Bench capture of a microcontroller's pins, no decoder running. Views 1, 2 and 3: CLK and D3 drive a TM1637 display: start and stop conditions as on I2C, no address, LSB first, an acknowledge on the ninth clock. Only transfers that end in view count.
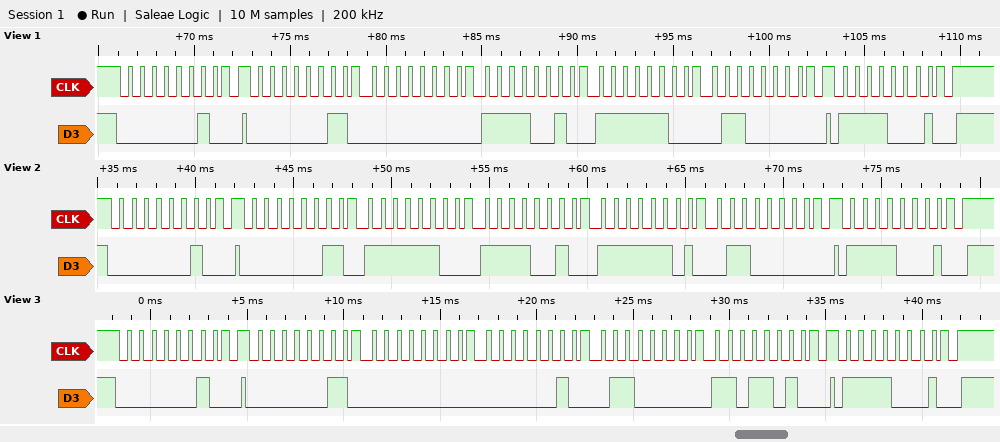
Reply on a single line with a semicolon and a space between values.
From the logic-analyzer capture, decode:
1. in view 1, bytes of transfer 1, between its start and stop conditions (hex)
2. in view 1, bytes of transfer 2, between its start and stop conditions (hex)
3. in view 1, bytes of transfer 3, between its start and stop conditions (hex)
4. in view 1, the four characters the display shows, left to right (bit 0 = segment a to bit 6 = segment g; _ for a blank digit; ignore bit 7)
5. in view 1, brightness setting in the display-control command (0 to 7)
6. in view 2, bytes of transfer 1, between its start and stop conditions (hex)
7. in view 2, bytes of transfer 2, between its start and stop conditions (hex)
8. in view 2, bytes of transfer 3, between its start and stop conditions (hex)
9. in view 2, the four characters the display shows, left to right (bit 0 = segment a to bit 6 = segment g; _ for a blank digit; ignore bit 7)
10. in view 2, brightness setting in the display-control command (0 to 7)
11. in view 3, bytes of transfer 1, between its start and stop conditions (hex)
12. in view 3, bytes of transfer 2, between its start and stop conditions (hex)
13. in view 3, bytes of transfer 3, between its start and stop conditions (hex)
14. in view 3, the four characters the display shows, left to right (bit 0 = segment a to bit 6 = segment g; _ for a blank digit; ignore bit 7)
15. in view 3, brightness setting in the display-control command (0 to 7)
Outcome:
40; C0 00 4F 3F 06; 8F; _301; 7; 40; C0 3F 4F BF 06; 8F; 0301; 7; 40; C0 00 40 06 5B; 8F; _-12; 7
